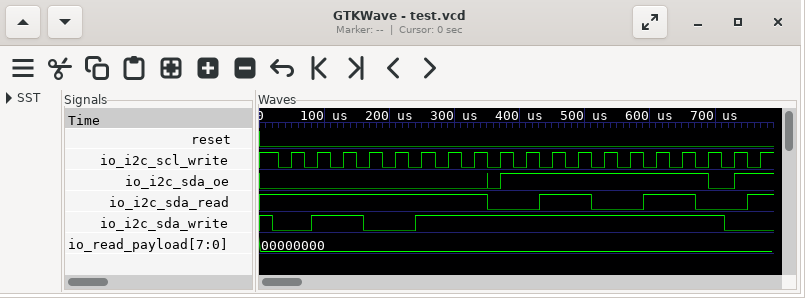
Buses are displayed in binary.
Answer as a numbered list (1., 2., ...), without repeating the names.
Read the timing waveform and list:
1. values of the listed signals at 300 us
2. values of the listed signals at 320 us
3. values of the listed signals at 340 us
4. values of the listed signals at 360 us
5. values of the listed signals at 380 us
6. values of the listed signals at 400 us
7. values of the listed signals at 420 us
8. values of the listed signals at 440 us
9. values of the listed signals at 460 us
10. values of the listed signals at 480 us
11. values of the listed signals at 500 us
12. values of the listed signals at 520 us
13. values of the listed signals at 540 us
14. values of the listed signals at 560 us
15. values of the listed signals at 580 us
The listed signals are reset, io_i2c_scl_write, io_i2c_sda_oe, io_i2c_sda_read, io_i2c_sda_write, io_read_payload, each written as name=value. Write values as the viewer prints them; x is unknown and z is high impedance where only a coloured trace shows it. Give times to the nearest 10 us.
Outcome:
1. reset=0, io_i2c_scl_write=1, io_i2c_sda_oe=0, io_i2c_sda_read=1, io_i2c_sda_write=1, io_read_payload=00000000
2. reset=0, io_i2c_scl_write=0, io_i2c_sda_oe=0, io_i2c_sda_read=1, io_i2c_sda_write=1, io_read_payload=00000000
3. reset=0, io_i2c_scl_write=1, io_i2c_sda_oe=0, io_i2c_sda_read=1, io_i2c_sda_write=1, io_read_payload=00000000
4. reset=0, io_i2c_scl_write=0, io_i2c_sda_oe=0, io_i2c_sda_read=0, io_i2c_sda_write=1, io_read_payload=00000000
5. reset=0, io_i2c_scl_write=1, io_i2c_sda_oe=1, io_i2c_sda_read=0, io_i2c_sda_write=1, io_read_payload=00000000
6. reset=0, io_i2c_scl_write=0, io_i2c_sda_oe=1, io_i2c_sda_read=0, io_i2c_sda_write=1, io_read_payload=00000000
7. reset=0, io_i2c_scl_write=1, io_i2c_sda_oe=1, io_i2c_sda_read=0, io_i2c_sda_write=1, io_read_payload=00000000
8. reset=0, io_i2c_scl_write=0, io_i2c_sda_oe=1, io_i2c_sda_read=1, io_i2c_sda_write=1, io_read_payload=00000000
9. reset=0, io_i2c_scl_write=1, io_i2c_sda_oe=1, io_i2c_sda_read=1, io_i2c_sda_write=1, io_read_payload=00000000
10. reset=0, io_i2c_scl_write=0, io_i2c_sda_oe=1, io_i2c_sda_read=1, io_i2c_sda_write=1, io_read_payload=00000000
11. reset=0, io_i2c_scl_write=1, io_i2c_sda_oe=1, io_i2c_sda_read=1, io_i2c_sda_write=1, io_read_payload=00000000
12. reset=0, io_i2c_scl_write=0, io_i2c_sda_oe=1, io_i2c_sda_read=0, io_i2c_sda_write=1, io_read_payload=00000000
13. reset=0, io_i2c_scl_write=1, io_i2c_sda_oe=1, io_i2c_sda_read=0, io_i2c_sda_write=1, io_read_payload=00000000
14. reset=0, io_i2c_scl_write=0, io_i2c_sda_oe=1, io_i2c_sda_read=0, io_i2c_sda_write=1, io_read_payload=00000000
15. reset=0, io_i2c_scl_write=1, io_i2c_sda_oe=1, io_i2c_sda_read=0, io_i2c_sda_write=1, io_read_payload=00000000
